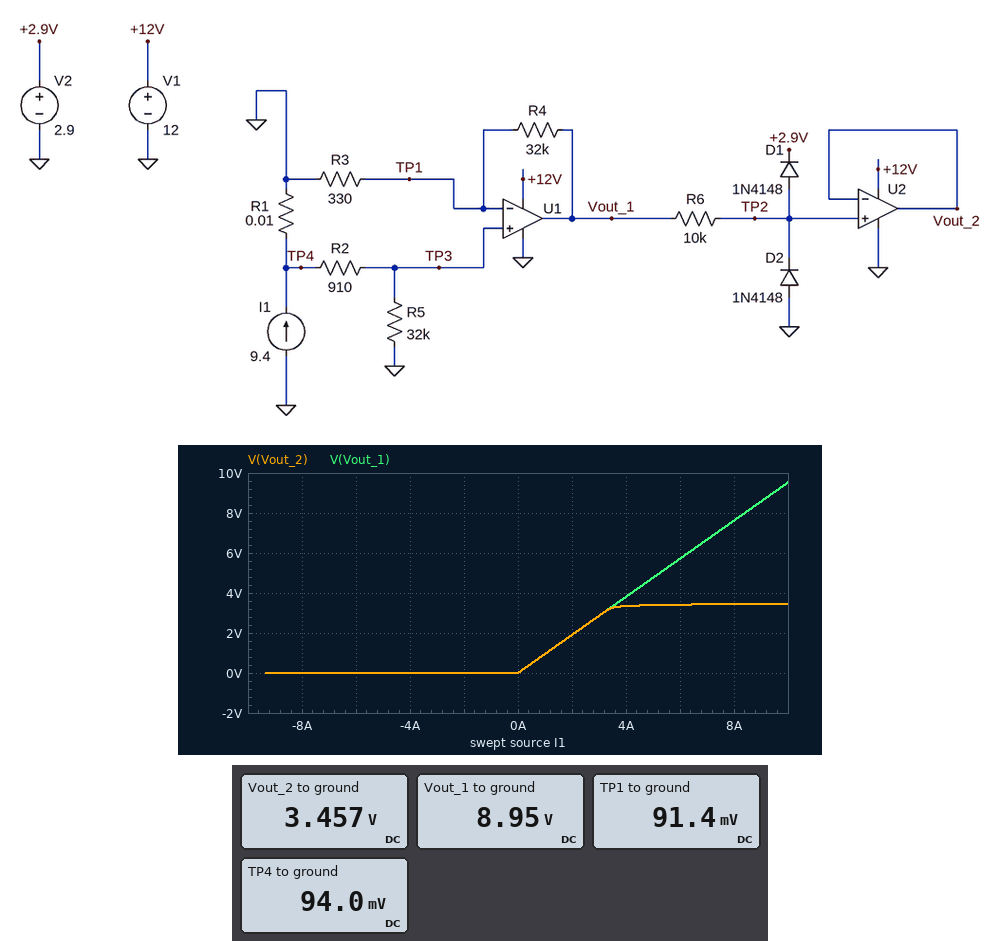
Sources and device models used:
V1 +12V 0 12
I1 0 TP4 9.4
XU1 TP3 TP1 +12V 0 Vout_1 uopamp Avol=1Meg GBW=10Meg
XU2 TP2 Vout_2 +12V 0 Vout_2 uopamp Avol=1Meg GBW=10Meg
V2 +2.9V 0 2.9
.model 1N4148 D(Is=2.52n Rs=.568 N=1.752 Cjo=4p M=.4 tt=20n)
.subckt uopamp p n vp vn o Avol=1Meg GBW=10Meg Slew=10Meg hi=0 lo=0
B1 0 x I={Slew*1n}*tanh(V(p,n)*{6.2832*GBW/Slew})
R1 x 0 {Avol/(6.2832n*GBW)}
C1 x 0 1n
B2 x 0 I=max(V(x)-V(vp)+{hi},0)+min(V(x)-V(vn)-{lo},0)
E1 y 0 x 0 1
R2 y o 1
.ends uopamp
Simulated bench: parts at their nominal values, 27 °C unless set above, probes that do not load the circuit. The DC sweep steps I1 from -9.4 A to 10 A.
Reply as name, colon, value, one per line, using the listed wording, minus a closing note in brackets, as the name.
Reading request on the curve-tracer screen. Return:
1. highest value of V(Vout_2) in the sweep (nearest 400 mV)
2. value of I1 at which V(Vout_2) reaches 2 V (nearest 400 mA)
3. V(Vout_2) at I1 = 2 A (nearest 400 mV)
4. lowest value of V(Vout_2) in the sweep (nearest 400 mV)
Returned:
highest value of V(Vout_2) in the sweep: 3.6 V
value of I1 at which V(Vout_2) reaches 2 V: 2.0 A
V(Vout_2) at I1 = 2 A: 2.0 V
lowest value of V(Vout_2) in the sweep: 0 V
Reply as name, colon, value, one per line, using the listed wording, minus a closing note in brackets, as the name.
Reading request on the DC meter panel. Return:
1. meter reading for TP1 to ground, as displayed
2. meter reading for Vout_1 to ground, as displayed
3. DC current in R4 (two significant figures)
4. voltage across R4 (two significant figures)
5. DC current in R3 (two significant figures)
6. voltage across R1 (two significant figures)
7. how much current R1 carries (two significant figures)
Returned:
meter reading for TP1 to ground, as displayed: 91.4 mV
meter reading for Vout_1 to ground, as displayed: 8.95 V
DC current in R4: 280 µA
voltage across R4: 8.9 V
DC current in R3: 280 µA
voltage across R1: 94 mV
how much current R1 carries: 9.4 A
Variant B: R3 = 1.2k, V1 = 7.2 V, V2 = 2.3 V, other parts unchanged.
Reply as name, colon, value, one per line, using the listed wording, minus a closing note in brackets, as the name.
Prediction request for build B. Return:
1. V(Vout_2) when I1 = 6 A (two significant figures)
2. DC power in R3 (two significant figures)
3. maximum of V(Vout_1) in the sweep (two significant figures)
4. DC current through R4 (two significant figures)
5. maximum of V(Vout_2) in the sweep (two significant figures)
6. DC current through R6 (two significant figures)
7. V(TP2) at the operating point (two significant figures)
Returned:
V(Vout_2) when I1 = 6 A: 1.6 V
DC power in R3: 7.0 µW
maximum of V(Vout_1) in the sweep: 2.7 V
DC current through R4: 76 µA
maximum of V(Vout_2) in the sweep: 2.6 V
DC current through R6: 360 nA
V(TP2) at the operating point: 2.5 V
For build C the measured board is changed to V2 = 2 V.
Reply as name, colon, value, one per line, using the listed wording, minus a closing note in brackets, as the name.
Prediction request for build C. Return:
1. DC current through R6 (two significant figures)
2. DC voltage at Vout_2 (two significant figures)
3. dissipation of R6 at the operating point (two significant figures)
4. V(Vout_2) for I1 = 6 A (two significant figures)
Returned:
DC current through R6: 640 µA
DC voltage at Vout_2: 2.6 V
dissipation of R6 at the operating point: 4.1 mW
V(Vout_2) for I1 = 6 A: 2.5 V
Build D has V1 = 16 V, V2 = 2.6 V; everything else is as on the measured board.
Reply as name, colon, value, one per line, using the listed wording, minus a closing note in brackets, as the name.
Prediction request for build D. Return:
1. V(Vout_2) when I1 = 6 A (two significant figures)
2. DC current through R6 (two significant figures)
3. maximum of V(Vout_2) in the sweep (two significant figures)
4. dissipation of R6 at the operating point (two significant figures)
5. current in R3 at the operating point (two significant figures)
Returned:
V(Vout_2) when I1 = 6 A: 3.1 V
DC current through R6: 580 µA
maximum of V(Vout_2) in the sweep: 3.2 V
dissipation of R6 at the operating point: 3.4 mW
current in R3 at the operating point: 280 µA
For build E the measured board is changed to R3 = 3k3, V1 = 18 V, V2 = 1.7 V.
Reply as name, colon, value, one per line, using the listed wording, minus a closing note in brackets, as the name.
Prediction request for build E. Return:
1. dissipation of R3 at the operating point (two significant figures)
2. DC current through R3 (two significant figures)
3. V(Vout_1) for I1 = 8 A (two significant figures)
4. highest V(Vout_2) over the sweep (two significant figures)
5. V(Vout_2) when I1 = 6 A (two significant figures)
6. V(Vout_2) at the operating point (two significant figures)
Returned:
dissipation of R3 at the operating point: 2.5 µW
DC current through R3: 28 µA
V(Vout_1) for I1 = 8 A: 830 mV
highest V(Vout_2) over the sweep: 1.0 V
V(Vout_2) when I1 = 6 A: 620 mV
V(Vout_2) at the operating point: 980 mV
